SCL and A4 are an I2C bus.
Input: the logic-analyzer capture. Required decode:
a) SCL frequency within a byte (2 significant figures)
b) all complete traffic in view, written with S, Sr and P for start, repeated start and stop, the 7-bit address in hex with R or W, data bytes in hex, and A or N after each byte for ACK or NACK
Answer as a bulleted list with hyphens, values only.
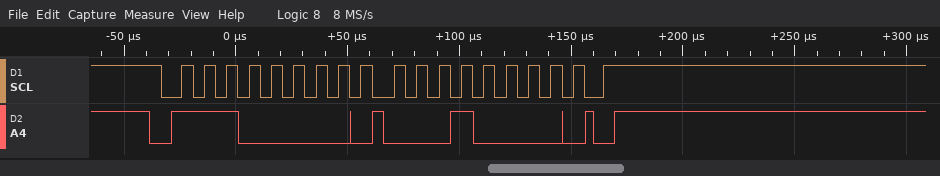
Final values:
- 100 kHz
- S 70W A 10 A P
